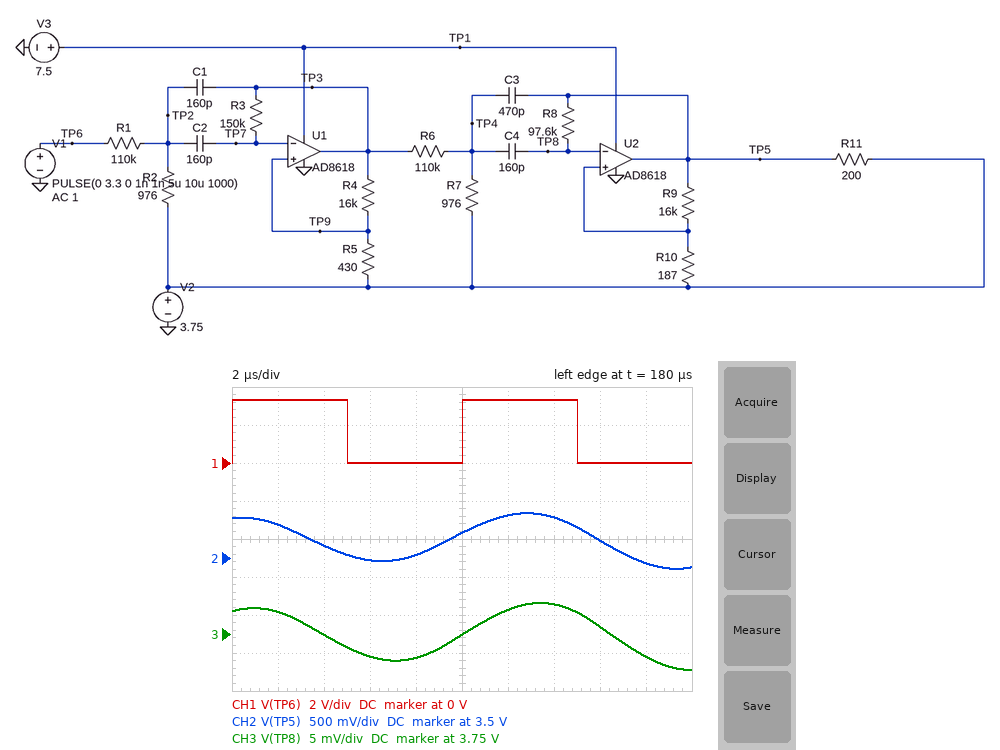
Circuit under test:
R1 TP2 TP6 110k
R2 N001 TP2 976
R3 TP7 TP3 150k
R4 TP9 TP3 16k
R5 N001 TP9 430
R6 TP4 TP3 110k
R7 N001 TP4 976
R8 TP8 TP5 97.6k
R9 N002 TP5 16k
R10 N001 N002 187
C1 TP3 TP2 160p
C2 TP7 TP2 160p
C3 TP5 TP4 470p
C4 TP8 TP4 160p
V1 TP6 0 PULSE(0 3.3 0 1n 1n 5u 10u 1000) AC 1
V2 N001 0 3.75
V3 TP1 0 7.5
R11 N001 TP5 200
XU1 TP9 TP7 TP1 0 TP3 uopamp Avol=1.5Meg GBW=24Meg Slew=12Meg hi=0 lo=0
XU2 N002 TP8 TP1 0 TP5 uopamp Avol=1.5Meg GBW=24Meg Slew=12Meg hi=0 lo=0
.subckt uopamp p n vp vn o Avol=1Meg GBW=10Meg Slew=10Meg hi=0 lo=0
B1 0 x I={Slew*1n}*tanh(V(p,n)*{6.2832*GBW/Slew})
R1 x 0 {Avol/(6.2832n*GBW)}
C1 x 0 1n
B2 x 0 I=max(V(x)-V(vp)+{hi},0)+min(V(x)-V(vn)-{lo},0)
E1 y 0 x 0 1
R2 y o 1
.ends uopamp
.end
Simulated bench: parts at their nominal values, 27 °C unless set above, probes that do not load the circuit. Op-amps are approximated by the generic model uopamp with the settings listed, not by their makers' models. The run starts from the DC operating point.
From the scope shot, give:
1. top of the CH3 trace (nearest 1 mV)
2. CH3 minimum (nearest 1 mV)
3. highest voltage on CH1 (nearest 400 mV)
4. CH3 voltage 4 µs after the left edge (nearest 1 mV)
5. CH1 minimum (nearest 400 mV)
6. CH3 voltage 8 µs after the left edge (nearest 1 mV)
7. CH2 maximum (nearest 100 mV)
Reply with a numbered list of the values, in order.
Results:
1. 3.754 V
2. 3.745 V
3. 3.2 V
4. 3.750 V
5. 0 V
6. 3.747 V
7. 4.1 V
